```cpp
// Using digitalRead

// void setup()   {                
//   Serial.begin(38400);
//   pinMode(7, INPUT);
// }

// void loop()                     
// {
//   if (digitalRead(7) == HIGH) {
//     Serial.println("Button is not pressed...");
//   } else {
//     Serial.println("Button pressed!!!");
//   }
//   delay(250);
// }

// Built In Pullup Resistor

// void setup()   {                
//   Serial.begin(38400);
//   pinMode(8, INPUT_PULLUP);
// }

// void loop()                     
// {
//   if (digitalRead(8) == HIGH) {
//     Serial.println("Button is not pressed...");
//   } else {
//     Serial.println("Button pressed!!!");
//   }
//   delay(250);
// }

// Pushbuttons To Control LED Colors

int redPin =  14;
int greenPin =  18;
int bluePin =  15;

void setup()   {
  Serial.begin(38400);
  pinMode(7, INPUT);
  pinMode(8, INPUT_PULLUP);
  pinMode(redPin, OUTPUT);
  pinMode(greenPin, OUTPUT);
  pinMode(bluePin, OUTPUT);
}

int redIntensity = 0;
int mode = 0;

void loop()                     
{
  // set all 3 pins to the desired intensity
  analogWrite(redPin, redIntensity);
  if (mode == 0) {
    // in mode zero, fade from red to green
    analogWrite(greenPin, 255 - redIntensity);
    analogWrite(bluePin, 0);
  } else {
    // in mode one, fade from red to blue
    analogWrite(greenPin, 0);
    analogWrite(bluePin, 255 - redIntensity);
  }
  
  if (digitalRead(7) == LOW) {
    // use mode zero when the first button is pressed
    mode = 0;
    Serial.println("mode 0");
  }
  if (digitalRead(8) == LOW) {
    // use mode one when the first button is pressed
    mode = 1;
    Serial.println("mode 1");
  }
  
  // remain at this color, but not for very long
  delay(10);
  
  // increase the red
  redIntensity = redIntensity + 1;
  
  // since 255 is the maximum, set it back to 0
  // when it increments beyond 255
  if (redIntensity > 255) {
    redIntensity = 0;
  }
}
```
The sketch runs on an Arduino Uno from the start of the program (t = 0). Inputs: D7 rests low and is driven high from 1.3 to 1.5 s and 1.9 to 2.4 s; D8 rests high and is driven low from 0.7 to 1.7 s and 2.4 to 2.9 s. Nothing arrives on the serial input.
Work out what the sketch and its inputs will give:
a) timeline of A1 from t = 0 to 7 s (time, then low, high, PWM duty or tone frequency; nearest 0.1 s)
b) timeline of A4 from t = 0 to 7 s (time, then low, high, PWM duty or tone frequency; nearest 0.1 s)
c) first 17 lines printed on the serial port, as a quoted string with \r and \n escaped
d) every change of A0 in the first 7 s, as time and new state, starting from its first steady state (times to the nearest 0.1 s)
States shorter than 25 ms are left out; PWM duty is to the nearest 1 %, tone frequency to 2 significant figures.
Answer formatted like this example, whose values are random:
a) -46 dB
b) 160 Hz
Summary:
a) 0 s low; 0.7 s high; 1.3 s low; 2.6 s high; 2.9 s low
b) 0 s high; 0.7 s low; 2.9 s high; 3.9 s low; 5.2 s high; 6.5 s low
c) "mode 0\r\nmode 0\r\nmode 0\r\nmode 0\r\nmode 0\r\nmode 0\r\nmode 0\r\nmode 0\r\nmode 0\r\nmode 0\r\nmode 0\r\nmode 0\r\nmode 0\r\nmode 0\r\nmode 0\r\nmode 0\r\nmode 0\r\n"
d) 0 s low; 1.3 s high; 2.6 s low; 3.9 s high; 5.2 s low; 6.5 s high
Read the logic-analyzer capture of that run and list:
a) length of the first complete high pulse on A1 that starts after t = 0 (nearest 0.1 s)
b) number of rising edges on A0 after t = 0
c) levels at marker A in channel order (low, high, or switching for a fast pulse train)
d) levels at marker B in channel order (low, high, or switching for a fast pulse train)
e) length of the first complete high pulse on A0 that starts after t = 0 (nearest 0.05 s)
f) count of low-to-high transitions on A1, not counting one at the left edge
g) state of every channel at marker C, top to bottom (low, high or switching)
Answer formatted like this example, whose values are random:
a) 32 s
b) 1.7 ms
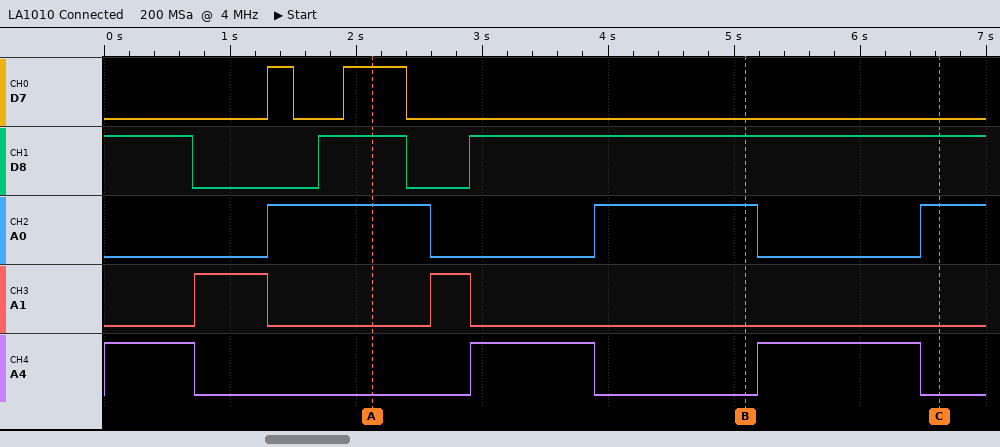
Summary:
a) 0.6 s
b) 3
c) D7 high, D8 high, A0 high, A1 low, A4 low
d) D7 low, D8 high, A0 high, A1 low, A4 low
e) 1.30 s
f) 2
g) D7 low, D8 high, A0 high, A1 low, A4 low
